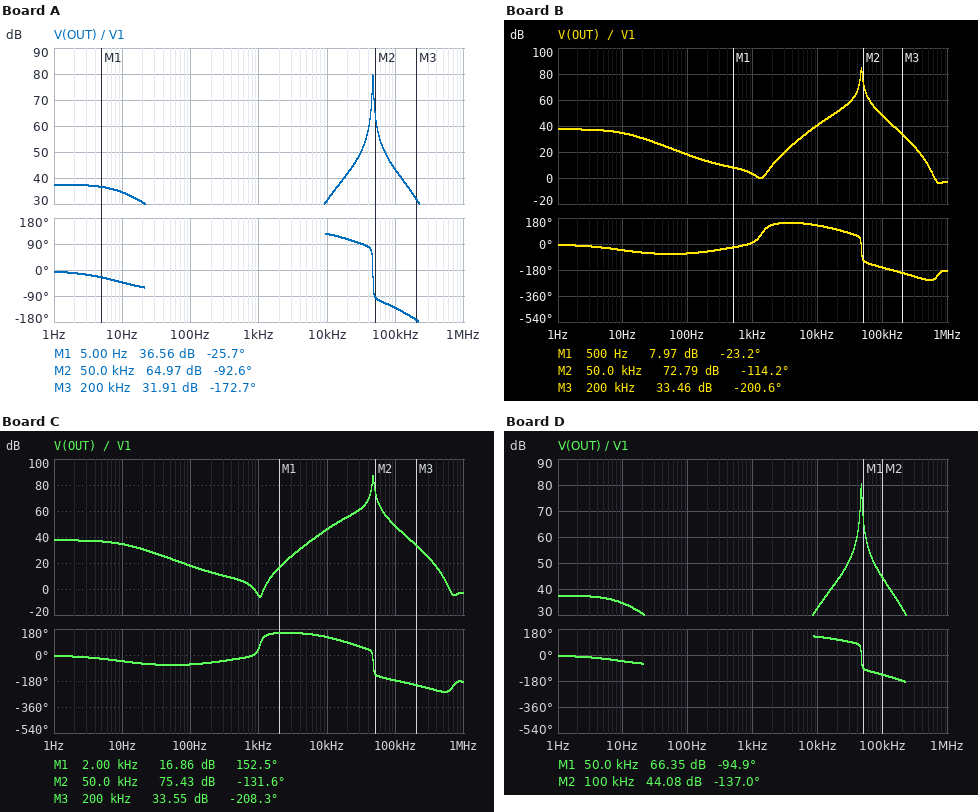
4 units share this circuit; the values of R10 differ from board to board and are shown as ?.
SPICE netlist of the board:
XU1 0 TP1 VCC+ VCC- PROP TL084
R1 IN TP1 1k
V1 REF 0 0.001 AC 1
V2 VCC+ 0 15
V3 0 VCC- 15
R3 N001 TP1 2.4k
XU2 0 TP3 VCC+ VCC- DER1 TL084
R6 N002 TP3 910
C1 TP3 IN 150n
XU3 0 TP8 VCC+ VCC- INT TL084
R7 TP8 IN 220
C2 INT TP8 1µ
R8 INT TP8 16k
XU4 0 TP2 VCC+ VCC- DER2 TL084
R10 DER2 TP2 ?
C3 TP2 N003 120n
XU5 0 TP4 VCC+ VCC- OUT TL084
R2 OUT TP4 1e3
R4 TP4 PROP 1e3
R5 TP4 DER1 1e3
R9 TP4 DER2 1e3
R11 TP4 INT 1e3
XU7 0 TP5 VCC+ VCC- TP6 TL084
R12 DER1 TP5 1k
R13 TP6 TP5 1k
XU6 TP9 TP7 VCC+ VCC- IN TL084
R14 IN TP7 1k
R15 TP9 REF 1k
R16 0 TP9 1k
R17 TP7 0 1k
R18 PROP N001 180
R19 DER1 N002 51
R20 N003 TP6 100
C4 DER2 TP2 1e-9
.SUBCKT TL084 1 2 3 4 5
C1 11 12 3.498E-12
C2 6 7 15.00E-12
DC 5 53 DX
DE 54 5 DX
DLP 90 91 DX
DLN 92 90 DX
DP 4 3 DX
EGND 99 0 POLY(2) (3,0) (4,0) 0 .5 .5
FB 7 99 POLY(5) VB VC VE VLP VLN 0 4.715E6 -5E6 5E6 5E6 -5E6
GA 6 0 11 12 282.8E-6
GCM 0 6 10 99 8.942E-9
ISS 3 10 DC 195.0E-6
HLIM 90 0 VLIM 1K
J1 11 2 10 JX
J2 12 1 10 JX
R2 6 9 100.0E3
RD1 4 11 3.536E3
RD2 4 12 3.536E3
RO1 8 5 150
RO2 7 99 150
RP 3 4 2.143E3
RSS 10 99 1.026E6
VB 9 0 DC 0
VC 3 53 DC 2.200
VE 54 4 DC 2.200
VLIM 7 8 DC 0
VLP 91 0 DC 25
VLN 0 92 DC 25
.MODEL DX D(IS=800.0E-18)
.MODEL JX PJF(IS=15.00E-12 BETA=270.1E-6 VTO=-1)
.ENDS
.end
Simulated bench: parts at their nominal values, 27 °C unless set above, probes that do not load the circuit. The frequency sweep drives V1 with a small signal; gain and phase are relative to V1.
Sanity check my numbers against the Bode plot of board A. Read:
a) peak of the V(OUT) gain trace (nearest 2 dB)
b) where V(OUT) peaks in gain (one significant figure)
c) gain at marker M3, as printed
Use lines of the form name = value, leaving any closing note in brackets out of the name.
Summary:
peak of the V(OUT) gain trace = 80 dB
where V(OUT) peaks in gain = 50 kHz
gain at marker M3, as printed = 31.91 dB
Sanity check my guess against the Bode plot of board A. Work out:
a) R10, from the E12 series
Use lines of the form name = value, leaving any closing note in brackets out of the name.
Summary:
R10, from the E12 series = 560 Ω
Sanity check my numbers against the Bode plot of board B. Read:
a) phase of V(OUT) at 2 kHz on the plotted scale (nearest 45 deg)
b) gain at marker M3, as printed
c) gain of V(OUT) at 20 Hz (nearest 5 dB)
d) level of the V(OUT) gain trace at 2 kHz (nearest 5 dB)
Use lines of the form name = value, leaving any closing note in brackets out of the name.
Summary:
phase of V(OUT) at 2 kHz on the plotted scale = 135 deg
gain at marker M3, as printed = 33.46 dB
gain of V(OUT) at 20 Hz = 30 dB
level of the V(OUT) gain trace at 2 kHz = 10 dB
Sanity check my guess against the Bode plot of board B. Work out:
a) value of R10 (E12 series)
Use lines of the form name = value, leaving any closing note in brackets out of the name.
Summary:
value of R10 = 1.8 kΩ
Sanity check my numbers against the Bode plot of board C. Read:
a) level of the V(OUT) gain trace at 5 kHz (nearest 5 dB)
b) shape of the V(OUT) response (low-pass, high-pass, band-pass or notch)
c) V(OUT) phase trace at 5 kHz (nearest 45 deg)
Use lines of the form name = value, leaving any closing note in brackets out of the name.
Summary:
level of the V(OUT) gain trace at 5 kHz = 35 dB
shape of the V(OUT) response = band-pass
V(OUT) phase trace at 5 kHz = 135 deg
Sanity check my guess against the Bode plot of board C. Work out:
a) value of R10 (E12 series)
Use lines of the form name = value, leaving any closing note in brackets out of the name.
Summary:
value of R10 = 3.3 kΩ
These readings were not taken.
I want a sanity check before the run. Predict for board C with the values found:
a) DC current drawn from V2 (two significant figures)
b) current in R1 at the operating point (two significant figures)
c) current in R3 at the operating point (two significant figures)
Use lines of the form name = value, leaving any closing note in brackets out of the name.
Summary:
DC current drawn from V2 = 99 mA
current in R1 at the operating point = 1.0 µA
current in R3 at the operating point = 1.0 µA
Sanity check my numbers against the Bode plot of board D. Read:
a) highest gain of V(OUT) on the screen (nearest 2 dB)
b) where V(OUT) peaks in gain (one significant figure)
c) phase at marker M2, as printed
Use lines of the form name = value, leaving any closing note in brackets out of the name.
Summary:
highest gain of V(OUT) on the screen = 80 dB
where V(OUT) peaks in gain = 50 kHz
phase at marker M2, as printed = -137.0 deg
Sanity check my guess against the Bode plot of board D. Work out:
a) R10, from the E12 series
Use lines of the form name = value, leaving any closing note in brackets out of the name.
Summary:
R10, from the E12 series = 680 Ω
